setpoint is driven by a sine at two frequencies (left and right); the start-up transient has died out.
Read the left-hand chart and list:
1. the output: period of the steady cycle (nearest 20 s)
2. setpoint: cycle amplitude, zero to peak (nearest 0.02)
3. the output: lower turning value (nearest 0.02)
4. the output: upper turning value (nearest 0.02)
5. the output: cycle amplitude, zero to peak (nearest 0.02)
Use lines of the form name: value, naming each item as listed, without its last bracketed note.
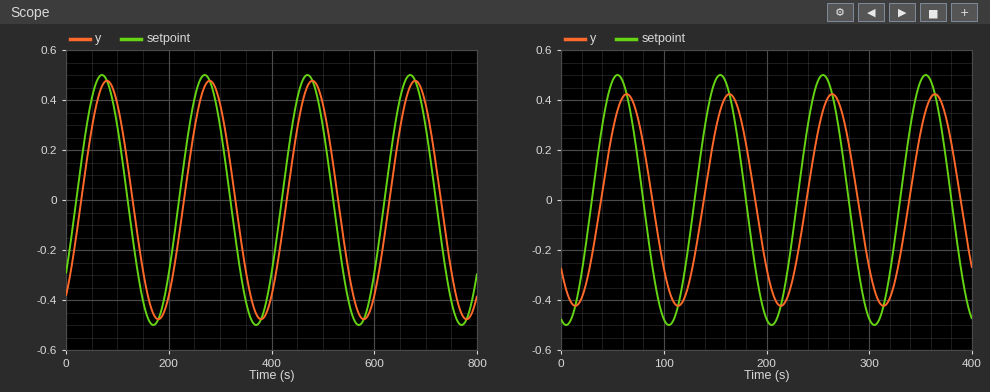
the output: period of the steady cycle: 200 s
setpoint: cycle amplitude, zero to peak: 0.50
the output: lower turning value: -0.48
the output: upper turning value: 0.48
the output: cycle amplitude, zero to peak: 0.48
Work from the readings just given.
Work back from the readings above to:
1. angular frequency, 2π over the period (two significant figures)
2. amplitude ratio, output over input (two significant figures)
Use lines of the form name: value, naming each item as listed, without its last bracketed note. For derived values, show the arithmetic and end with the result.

angular frequency, 2π over the period: 2π / 200 = 0.031 rad/s
amplitude ratio, output over input: 0.48 / 0.5 = 0.96
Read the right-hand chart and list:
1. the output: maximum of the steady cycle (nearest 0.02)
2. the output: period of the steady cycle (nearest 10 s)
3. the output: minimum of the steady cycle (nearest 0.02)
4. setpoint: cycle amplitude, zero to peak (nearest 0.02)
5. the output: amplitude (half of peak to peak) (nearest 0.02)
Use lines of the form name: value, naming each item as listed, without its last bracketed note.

the output: maximum of the steady cycle: 0.42
the output: period of the steady cycle: 100 s
the output: minimum of the steady cycle: -0.42
setpoint: cycle amplitude, zero to peak: 0.50
the output: amplitude (half of peak to peak): 0.42
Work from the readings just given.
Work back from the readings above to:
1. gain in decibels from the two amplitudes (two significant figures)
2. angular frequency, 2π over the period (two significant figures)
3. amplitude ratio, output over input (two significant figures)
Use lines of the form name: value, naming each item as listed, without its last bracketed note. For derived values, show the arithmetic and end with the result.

gain in decibels from the two amplitudes: 20 log10(0.42 / 0.5) = -1.5 dB
angular frequency, 2π over the period: 2π / 100 = 0.063 rad/s
amplitude ratio, output over input: 0.42 / 0.5 = 0.84
